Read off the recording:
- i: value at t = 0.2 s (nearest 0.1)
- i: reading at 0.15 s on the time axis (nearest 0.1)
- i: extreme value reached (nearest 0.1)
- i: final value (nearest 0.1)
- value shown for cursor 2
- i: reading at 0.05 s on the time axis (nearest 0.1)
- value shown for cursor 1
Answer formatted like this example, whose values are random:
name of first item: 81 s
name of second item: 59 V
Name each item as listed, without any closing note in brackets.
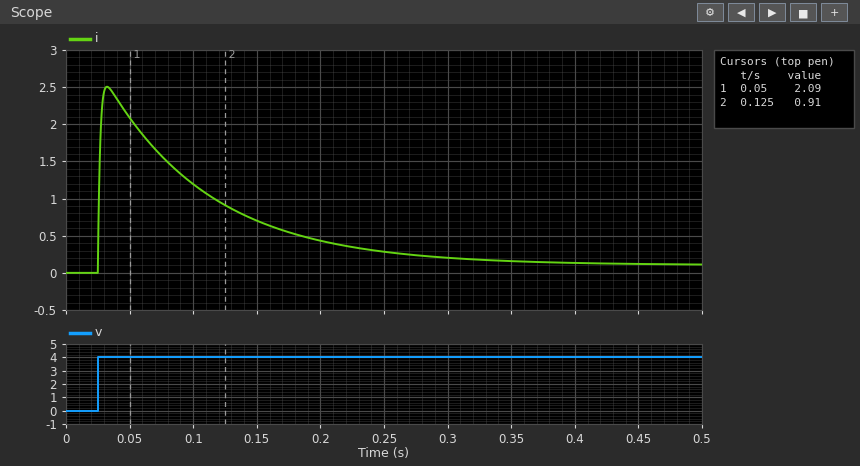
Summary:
i: value at t = 0.2 s: 0.4
i: reading at 0.15 s on the time axis: 0.7
i: extreme value reached: 2.5
i: final value: 0.1
value shown for cursor 2: 0.91
i: reading at 0.05 s on the time axis: 2.1
value shown for cursor 1: 2.09
